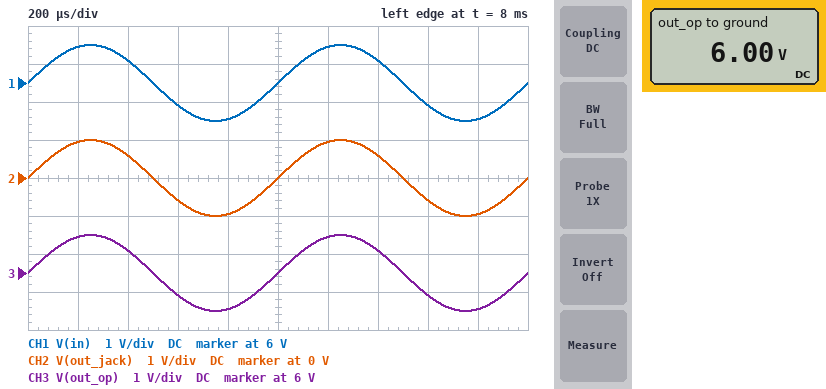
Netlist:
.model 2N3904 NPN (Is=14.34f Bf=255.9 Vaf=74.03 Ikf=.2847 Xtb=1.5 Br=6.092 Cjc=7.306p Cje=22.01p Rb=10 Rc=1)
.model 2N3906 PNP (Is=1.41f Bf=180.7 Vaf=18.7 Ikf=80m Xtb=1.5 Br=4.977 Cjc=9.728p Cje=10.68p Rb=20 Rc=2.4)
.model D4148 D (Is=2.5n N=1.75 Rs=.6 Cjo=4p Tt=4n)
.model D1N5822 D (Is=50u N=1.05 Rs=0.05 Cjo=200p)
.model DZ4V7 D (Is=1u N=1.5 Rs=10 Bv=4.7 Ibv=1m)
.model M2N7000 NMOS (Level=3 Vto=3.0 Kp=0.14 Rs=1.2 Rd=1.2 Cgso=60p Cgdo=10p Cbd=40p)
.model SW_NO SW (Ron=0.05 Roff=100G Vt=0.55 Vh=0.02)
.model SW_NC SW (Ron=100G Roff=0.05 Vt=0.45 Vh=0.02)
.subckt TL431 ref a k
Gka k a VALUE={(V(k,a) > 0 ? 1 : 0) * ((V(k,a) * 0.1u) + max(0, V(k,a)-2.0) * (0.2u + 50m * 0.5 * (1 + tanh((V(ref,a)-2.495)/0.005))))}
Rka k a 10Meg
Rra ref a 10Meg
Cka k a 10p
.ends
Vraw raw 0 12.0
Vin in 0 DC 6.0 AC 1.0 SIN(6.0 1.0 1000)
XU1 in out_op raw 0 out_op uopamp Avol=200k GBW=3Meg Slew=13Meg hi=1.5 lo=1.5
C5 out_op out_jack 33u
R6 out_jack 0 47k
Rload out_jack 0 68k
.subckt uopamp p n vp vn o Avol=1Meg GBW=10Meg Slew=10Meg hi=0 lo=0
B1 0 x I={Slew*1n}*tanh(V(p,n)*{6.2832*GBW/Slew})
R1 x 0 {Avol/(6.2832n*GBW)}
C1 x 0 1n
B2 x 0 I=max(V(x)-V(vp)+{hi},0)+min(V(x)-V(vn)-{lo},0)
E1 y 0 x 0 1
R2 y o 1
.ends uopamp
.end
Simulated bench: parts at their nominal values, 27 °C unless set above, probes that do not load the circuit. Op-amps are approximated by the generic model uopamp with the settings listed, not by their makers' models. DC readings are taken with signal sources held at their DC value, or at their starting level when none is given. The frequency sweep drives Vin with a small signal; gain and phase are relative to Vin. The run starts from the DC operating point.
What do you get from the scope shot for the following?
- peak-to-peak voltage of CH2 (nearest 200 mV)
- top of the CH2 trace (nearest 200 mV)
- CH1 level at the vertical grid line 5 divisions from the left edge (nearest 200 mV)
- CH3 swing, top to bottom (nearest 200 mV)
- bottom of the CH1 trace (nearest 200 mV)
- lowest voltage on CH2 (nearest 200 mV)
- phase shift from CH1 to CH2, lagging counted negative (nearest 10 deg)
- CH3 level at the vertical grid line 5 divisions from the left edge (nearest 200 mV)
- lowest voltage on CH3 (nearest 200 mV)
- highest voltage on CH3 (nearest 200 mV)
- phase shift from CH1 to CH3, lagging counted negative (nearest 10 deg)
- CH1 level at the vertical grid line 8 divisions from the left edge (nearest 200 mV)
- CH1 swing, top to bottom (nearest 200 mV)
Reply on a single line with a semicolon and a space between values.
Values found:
2.0 V; 1.0 V; 6.0 V; 2.0 V; 5.0 V; -1.0 V; 0 deg; 6.0 V; 5.0 V; 7.0 V; 0 deg; 5.4 V; 2.0 V
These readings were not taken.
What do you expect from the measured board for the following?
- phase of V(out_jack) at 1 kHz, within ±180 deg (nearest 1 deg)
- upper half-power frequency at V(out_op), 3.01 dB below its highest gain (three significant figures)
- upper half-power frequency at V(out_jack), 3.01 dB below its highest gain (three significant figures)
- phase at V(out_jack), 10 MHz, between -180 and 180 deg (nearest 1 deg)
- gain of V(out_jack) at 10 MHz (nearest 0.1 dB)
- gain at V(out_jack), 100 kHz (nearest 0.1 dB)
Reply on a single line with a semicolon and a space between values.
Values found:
0 deg; 3.00 MHz; 3.00 MHz; -73 deg; -10.8 dB; 0 dB
